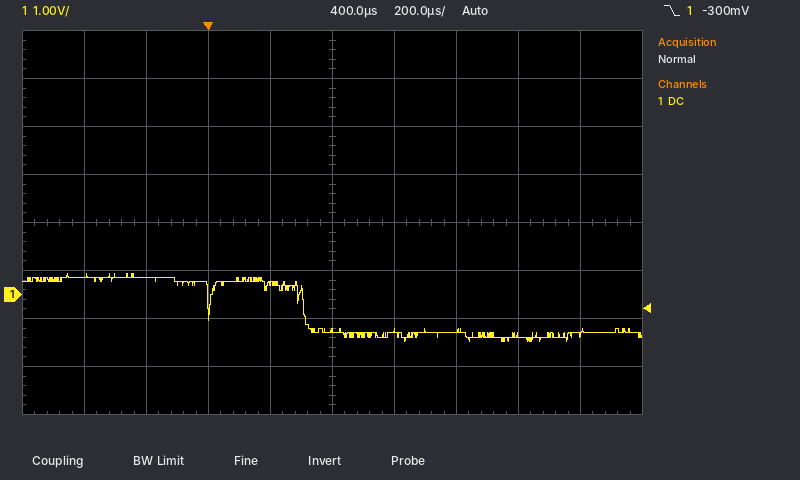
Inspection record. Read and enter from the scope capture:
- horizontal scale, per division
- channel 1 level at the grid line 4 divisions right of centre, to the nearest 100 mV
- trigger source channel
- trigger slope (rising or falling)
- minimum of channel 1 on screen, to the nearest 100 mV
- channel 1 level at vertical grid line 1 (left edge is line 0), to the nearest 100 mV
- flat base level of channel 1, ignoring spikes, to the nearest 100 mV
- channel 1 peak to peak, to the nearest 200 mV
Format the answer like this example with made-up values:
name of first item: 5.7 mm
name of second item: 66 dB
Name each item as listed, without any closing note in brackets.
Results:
horizontal scale, per division: 200 µs
channel 1 level at the grid line 4 divisions right of centre, to the nearest 100 mV: -800 mV
trigger source channel: channel 1
trigger slope: falling
minimum of channel 1 on screen, to the nearest 100 mV: -1.0 V
channel 1 level at vertical grid line 1 (left edge is line 0), to the nearest 100 mV: 400 mV
flat base level of channel 1, ignoring spikes, to the nearest 100 mV: -800 mV
channel 1 peak to peak, to the nearest 200 mV: 1.4 V
